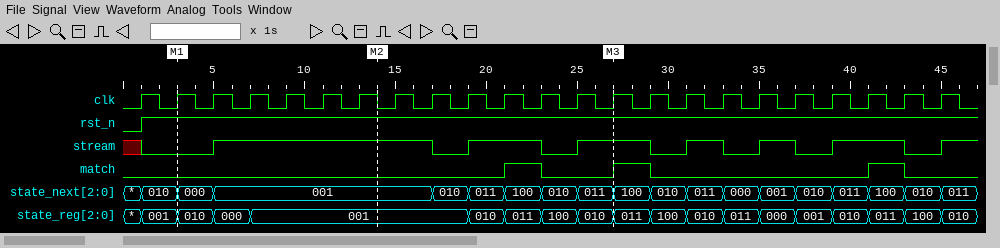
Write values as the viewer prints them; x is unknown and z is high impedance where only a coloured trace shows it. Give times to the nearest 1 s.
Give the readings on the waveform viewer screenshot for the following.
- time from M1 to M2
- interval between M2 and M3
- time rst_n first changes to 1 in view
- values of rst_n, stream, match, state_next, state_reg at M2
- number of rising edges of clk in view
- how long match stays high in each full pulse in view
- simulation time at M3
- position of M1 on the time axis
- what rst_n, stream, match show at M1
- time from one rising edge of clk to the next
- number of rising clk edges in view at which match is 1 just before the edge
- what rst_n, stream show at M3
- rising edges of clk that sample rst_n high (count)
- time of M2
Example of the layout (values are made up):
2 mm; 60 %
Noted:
11 s; 13 s; 1 s; rst_n=1, stream=1, match=0, state_next=001, state_reg=001; 23; 2 s, 2 s, 2 s; 27 s; 3 s; rst_n=1, stream=0, match=0; 2 s; 3; rst_n=1, stream=1; 22; 14 s
